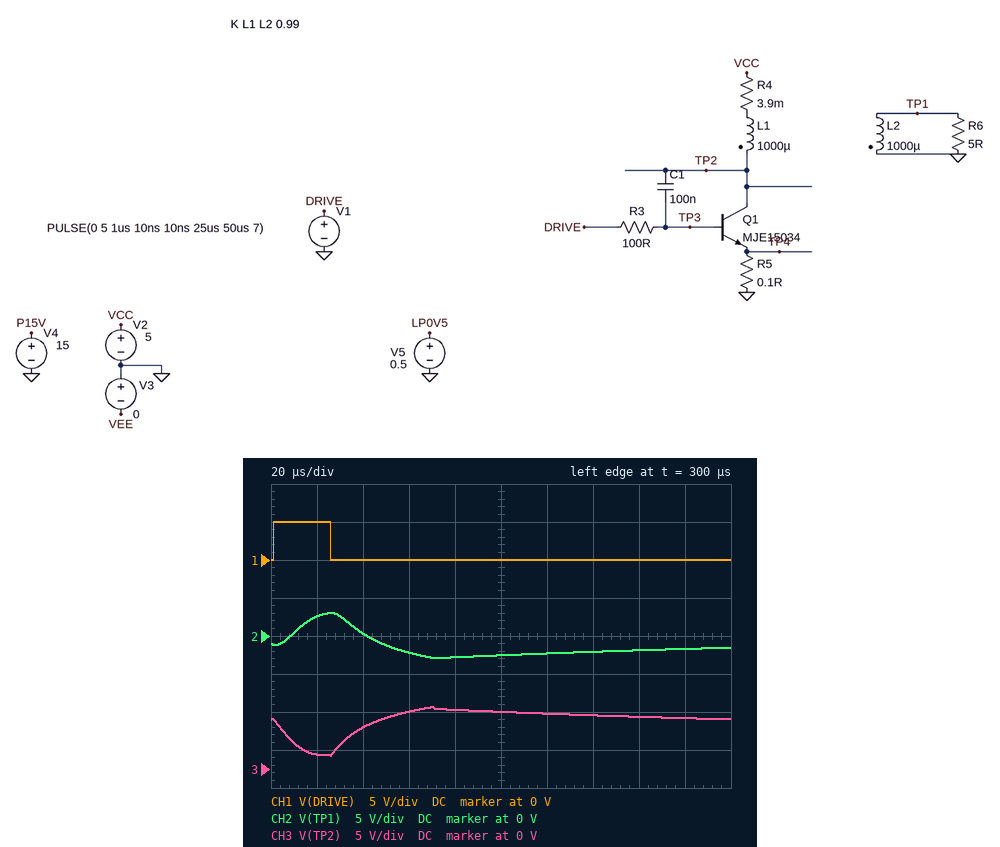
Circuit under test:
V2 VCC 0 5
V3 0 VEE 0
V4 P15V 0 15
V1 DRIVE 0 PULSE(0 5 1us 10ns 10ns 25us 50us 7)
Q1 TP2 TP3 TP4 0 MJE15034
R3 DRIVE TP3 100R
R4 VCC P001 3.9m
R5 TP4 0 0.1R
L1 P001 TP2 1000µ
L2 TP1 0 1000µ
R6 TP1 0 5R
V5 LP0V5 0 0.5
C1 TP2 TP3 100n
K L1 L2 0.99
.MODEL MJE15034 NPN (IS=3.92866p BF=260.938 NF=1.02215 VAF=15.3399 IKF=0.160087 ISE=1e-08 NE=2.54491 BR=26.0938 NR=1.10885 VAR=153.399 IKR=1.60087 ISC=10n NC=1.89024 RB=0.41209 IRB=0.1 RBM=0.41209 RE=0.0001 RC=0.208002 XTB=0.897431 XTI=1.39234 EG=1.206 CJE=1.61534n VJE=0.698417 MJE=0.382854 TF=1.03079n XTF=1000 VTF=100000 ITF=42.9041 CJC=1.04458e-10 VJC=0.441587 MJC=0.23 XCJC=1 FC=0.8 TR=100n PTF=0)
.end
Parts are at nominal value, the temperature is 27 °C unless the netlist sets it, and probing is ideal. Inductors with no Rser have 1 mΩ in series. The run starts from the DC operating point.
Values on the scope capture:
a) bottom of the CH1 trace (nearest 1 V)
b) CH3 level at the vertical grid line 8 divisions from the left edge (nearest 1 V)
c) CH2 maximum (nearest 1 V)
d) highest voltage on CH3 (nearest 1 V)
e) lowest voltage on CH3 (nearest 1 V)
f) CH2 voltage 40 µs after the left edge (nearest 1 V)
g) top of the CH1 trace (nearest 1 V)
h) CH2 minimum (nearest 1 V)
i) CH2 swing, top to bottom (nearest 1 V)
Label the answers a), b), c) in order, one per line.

a) 0 V
b) 7 V
c) 3 V
d) 8 V
e) 2 V
f) 0 V
g) 5 V
h) -3 V
i) 6 V
